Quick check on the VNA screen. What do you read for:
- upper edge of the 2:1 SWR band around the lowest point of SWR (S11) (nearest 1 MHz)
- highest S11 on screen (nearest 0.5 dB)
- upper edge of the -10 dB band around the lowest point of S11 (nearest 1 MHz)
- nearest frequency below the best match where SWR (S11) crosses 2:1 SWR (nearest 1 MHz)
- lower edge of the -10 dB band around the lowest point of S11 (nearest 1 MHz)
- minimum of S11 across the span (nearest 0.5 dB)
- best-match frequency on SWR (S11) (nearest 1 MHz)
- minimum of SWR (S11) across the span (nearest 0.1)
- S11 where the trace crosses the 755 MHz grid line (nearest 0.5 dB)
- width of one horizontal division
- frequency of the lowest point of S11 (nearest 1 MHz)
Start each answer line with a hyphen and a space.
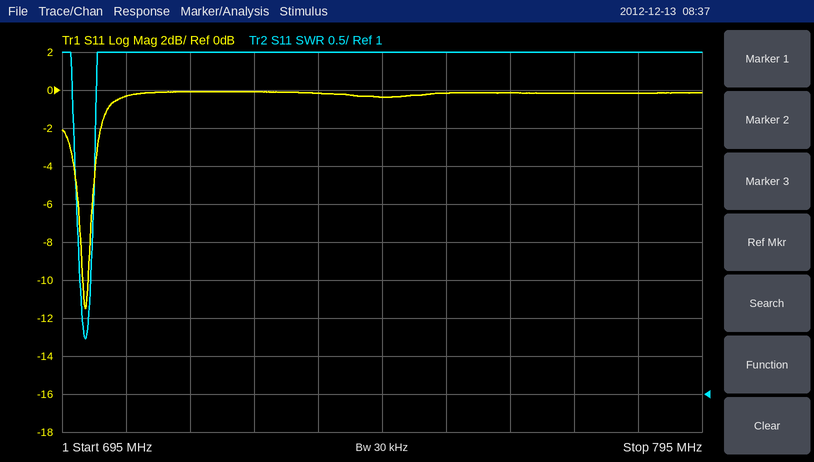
- 699 MHz
- 0.0 dB
- 699 MHz
- 698 MHz
- 698 MHz
- -11.5 dB
- 699 MHz
- 1.7
- 0.0 dB
- 10 MHz
- 699 MHz
